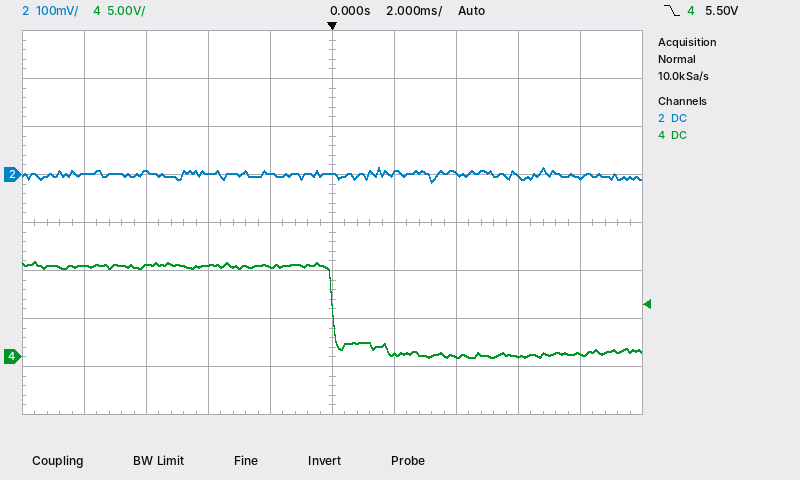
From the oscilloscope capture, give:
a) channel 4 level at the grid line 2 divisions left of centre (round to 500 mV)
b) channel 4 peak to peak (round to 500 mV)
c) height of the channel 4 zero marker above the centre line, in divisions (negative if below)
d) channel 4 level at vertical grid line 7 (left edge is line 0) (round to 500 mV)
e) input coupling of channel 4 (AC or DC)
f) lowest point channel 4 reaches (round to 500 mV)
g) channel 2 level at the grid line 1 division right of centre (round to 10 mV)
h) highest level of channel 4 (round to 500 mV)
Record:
9.5 V
10.0 V
-2.8 div
0.0 V
DC
0.0 V
0 mV
10.0 V
